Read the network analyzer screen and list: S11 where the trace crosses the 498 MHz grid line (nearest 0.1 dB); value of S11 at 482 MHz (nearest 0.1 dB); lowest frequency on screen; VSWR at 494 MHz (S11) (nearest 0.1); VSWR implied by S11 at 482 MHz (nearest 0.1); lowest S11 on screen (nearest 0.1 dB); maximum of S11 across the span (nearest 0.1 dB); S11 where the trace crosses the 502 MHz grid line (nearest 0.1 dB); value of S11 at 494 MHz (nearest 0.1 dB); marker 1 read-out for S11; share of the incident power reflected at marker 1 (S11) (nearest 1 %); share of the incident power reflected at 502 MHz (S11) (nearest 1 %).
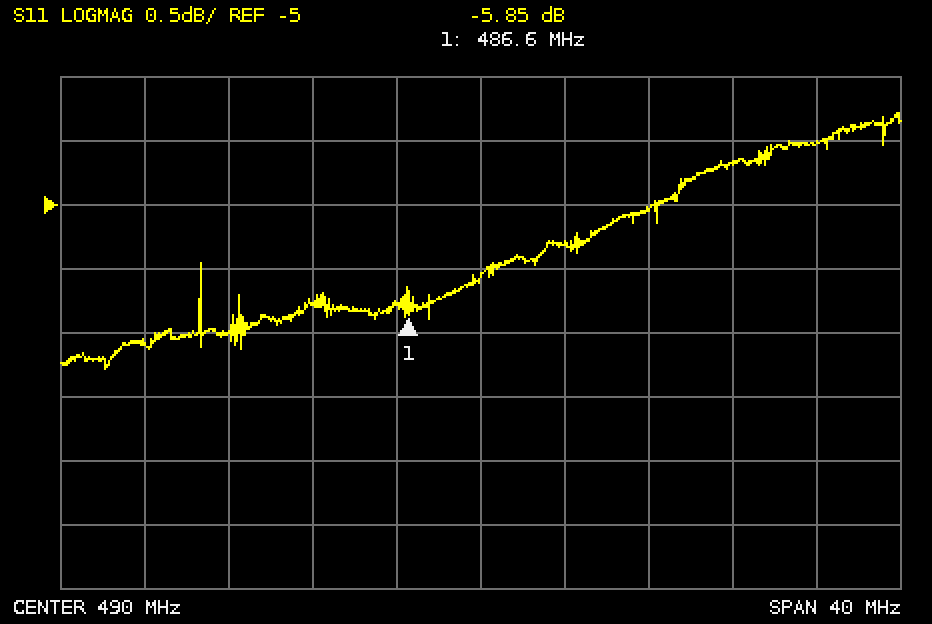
-5.0 dB
-5.8 dB
470 MHz
3.4
3.1
-6.3 dB
-4.3 dB
-4.7 dB
-5.3 dB
-5.85 dB
26 %
34 %
